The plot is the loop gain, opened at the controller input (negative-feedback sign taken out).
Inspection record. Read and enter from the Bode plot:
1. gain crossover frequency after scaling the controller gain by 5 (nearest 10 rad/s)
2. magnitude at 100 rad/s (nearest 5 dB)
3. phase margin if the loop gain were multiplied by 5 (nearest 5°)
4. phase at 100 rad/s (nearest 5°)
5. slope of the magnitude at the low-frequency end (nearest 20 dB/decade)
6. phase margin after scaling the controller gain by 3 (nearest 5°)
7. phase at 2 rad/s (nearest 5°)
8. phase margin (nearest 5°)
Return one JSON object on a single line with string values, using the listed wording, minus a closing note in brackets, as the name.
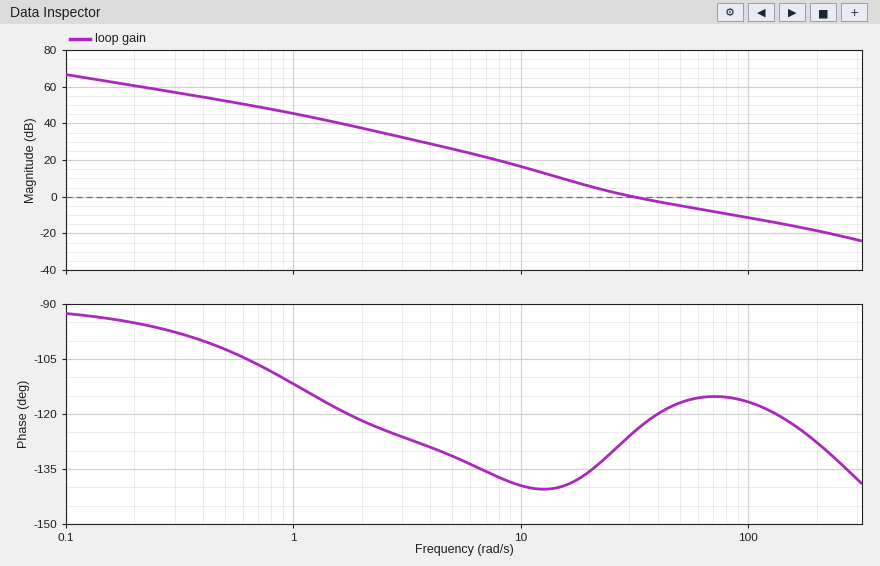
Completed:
{"gain crossover frequency after scaling the controller gain by 5": "130 rad/s", "magnitude at 100 rad/s": "-10 dB", "phase margin if the loop gain were multiplied by 5": "60°", "phase at 100 rad/s": "-115°", "slope of the magnitude at the low-frequency end": "-20 dB/decade", "phase margin after scaling the controller gain by 3": "65°", "phase at 2 rad/s": "-120°", "phase margin": "55°"}
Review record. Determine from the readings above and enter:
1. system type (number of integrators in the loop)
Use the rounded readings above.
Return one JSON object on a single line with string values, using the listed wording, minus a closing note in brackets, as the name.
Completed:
{"system type": "1"}
